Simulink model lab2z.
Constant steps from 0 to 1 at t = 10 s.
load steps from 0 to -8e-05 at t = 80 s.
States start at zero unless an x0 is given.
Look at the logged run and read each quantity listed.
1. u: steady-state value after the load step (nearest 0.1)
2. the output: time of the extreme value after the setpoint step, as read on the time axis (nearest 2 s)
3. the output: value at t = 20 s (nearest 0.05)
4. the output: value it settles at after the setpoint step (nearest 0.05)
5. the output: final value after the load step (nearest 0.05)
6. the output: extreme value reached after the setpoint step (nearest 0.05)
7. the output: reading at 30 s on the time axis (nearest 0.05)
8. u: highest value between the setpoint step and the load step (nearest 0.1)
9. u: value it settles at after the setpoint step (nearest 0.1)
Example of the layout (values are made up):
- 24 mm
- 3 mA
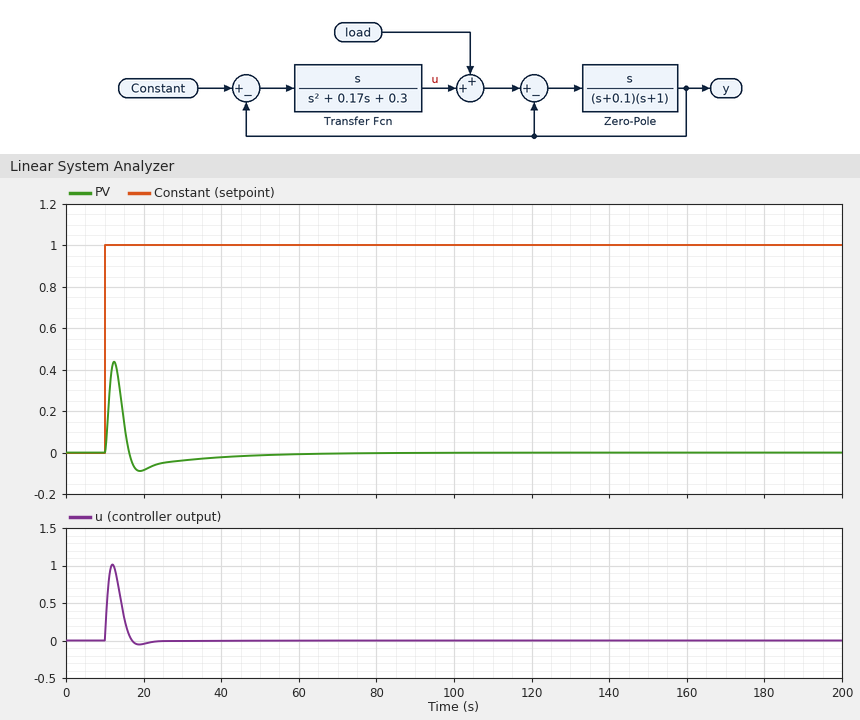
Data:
- 0.0
- 12 s
- -0.10
- 0.00
- 0.00
- 0.45
- -0.05
- 1.0
- 0.0
